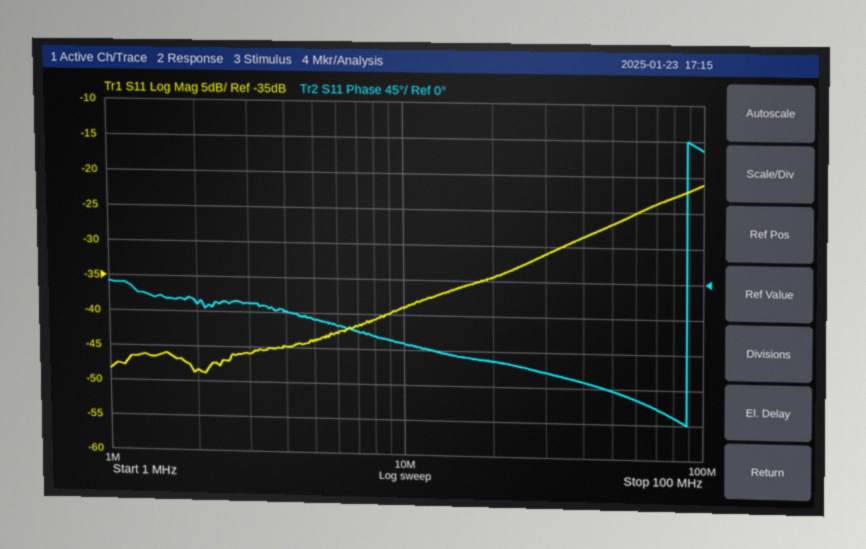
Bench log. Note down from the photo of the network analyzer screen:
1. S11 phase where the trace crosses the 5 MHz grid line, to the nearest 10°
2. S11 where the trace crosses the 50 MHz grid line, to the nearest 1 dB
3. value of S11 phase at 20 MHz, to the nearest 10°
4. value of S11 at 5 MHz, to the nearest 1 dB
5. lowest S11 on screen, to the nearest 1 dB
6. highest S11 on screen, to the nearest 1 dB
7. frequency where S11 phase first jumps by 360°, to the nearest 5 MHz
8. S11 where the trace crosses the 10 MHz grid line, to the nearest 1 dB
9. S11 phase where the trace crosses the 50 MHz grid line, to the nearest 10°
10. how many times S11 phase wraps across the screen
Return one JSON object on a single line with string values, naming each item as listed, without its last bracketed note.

{"S11 phase where the trace crosses the 5 MHz grid line, to the nearest 10°": "-50°", "S11 where the trace crosses the 50 MHz grid line, to the nearest 1 dB": "-27 dB", "value of S11 phase at 20 MHz, to the nearest 10°": "-100°", "value of S11 at 5 MHz, to the nearest 1 dB": "-44 dB", "lowest S11 on screen, to the nearest 1 dB": "-49 dB", "highest S11 on screen, to the nearest 1 dB": "-21 dB", "frequency where S11 phase first jumps by 360°, to the nearest 5 MHz": "90 MHz", "S11 where the trace crosses the 10 MHz grid line, to the nearest 1 dB": "-39 dB", "S11 phase where the trace crosses the 50 MHz grid line, to the nearest 10°": "-140°", "how many times S11 phase wraps across the screen": "1"}
